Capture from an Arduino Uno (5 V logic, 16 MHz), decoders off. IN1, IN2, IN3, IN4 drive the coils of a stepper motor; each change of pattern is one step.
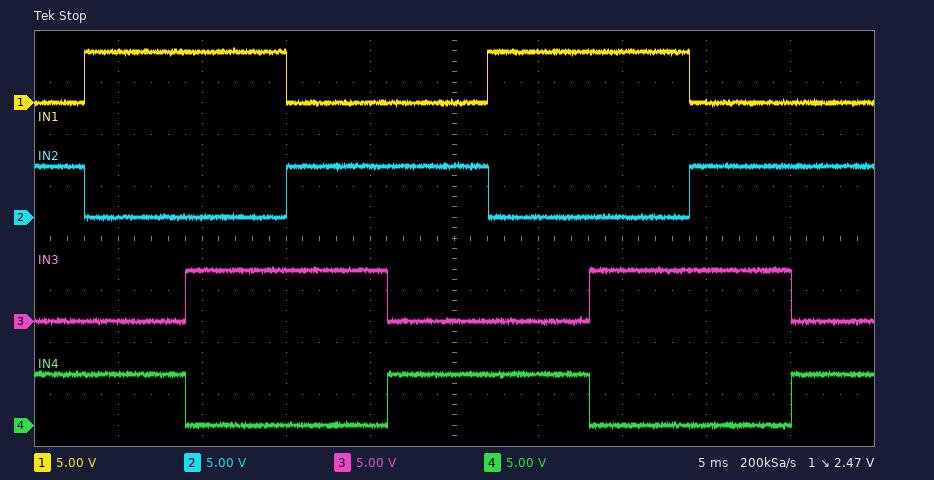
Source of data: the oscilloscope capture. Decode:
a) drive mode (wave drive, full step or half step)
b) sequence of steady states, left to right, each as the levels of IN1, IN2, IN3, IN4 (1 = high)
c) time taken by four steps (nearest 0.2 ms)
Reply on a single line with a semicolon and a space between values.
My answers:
full step; 0101 1001 1010 0110 0101 1001 1010 0110 0101; 24.0 ms
